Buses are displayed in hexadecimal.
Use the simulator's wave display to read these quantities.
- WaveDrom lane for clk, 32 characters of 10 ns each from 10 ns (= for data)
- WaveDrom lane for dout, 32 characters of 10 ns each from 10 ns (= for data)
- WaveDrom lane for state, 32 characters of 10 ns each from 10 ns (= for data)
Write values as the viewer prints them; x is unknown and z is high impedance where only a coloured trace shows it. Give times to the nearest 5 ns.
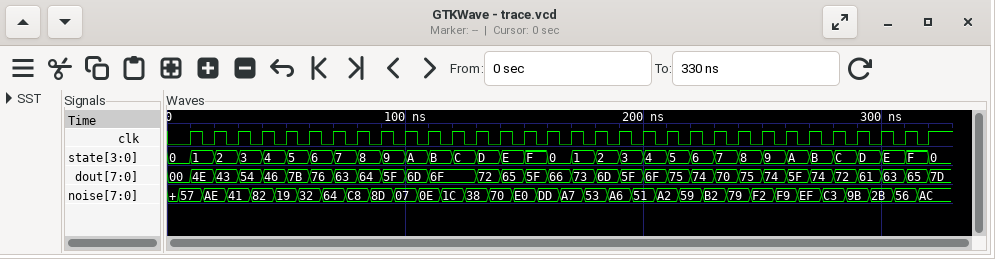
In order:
{name: 'clk', wave: 'p...............................'}
{name: 'dout', wave: '===========.====================', data: '4E 43 54 46 7B 76 63 64 5F 6D 6F 72 65 5F 66 73 6D 5F 6F 75 74 70 75 74 5F 74 72 61 63 65 7D'}
{name: 'state', wave: '================================', data: '1 2 3 4 5 6 7 8 9 A B C D E F 0 1 2 3 4 5 6 7 8 9 A B C D E F 0'}
